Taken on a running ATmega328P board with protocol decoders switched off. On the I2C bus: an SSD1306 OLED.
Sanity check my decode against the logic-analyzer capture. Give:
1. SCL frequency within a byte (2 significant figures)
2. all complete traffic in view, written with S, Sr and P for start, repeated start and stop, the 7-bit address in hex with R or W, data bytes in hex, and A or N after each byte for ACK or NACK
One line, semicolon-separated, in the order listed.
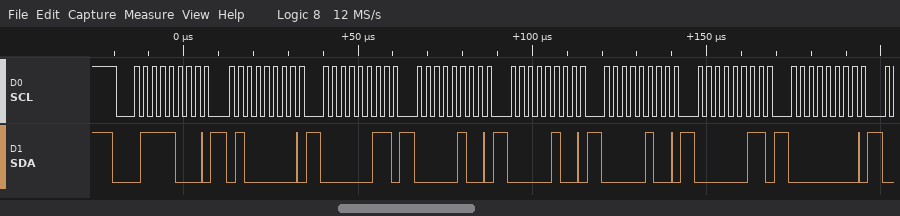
400 kHz; S 3CW A 40 A 03 A 04 A 04 A 04 A 03 A 00 A
